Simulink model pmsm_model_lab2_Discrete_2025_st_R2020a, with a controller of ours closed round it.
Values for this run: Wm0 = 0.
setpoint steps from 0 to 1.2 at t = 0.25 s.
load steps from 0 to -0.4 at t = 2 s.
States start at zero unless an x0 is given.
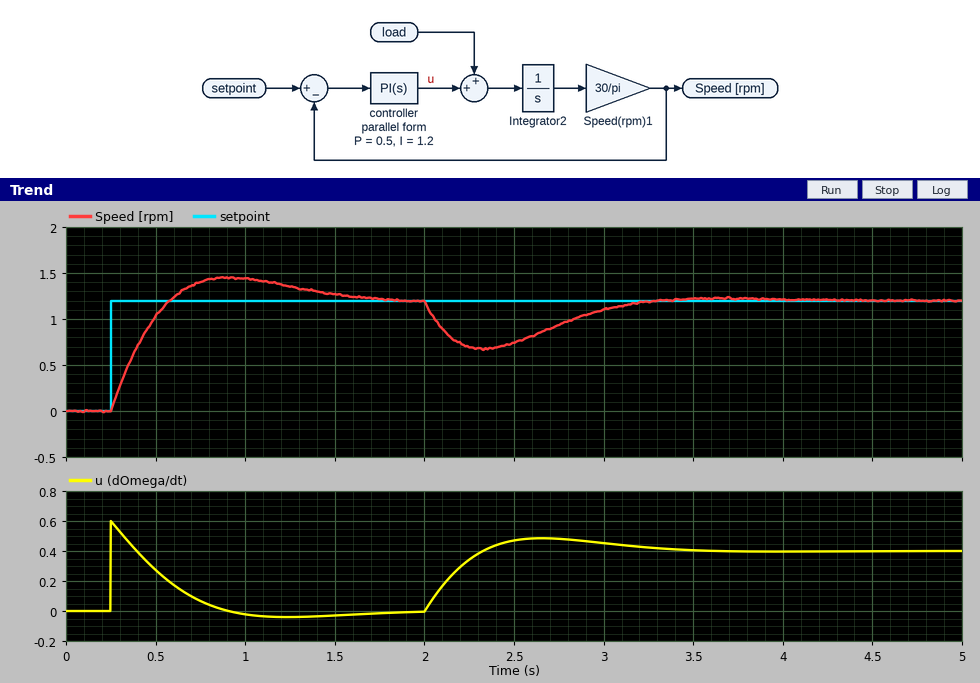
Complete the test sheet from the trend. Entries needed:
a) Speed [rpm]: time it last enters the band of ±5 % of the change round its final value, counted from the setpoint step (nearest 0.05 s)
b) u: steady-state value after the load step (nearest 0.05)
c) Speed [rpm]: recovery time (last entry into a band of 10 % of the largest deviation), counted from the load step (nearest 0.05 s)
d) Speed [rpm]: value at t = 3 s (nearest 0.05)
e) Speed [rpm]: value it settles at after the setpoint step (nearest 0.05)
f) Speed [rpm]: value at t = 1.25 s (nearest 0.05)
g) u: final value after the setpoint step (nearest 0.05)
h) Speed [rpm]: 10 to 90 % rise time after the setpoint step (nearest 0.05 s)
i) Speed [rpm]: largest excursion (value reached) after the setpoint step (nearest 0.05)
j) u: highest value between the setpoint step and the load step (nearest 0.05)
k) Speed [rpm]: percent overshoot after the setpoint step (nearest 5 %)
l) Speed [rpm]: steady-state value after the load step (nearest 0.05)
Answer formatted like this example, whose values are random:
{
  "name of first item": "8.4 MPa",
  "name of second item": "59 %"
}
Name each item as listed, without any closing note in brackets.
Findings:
{
  "Speed [rpm]: time it last enters the band of ±5 % of the change round its final value, counted from the setpoint step": "1.30 s",
  "u: steady-state value after the load step": "0.40",
  "Speed [rpm]: recovery time (last entry into a band of 10 % of the largest deviation), counted from the load step": "1.10 s",
  "Speed [rpm]: value at t = 3 s": "1.10",
  "Speed [rpm]: value it settles at after the setpoint step": "1.20",
  "Speed [rpm]: value at t = 1.25 s": "1.35",
  "u: final value after the setpoint step": "0.00",
  "Speed [rpm]: 10 to 90 % rise time after the setpoint step": "0.25 s",
  "Speed [rpm]: largest excursion (value reached) after the setpoint step": "1.45",
  "u: highest value between the setpoint step and the load step": "0.60",
  "Speed [rpm]: percent overshoot after the setpoint step": "20 %",
  "Speed [rpm]: steady-state value after the load step": "1.20"
}
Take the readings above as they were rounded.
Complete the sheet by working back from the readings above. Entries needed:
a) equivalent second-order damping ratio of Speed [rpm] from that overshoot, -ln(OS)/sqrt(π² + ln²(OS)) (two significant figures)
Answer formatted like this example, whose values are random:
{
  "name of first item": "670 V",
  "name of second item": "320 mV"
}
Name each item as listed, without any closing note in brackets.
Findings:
{
  "equivalent second-order damping ratio of Speed [rpm] from that overshoot, -ln(OS)/sqrt(π² + ln²(OS))": "0.46"
}
